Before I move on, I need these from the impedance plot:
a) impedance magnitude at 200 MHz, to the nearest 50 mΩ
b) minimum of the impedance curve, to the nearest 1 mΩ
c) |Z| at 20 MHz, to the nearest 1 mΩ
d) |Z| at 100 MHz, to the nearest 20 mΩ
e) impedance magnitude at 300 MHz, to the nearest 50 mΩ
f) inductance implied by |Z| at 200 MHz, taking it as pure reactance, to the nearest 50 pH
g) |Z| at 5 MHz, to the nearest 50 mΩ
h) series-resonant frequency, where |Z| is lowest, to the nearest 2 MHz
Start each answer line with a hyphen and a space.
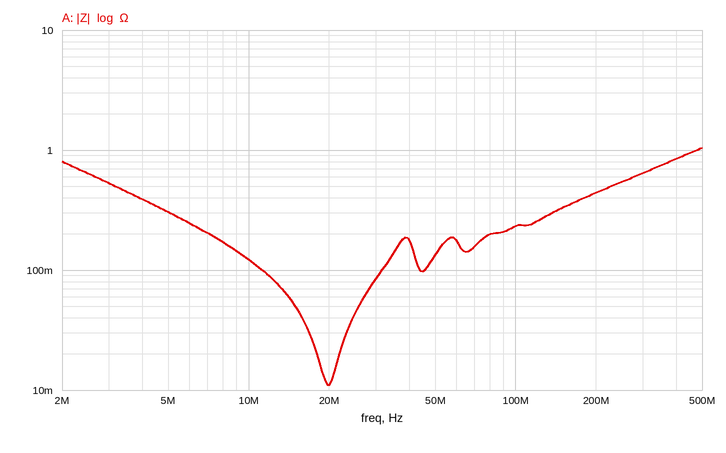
- 450 mΩ
- 11 mΩ
- 11 mΩ
- 240 mΩ
- 650 mΩ
- 350 pH
- 300 mΩ
- 20 MHz
